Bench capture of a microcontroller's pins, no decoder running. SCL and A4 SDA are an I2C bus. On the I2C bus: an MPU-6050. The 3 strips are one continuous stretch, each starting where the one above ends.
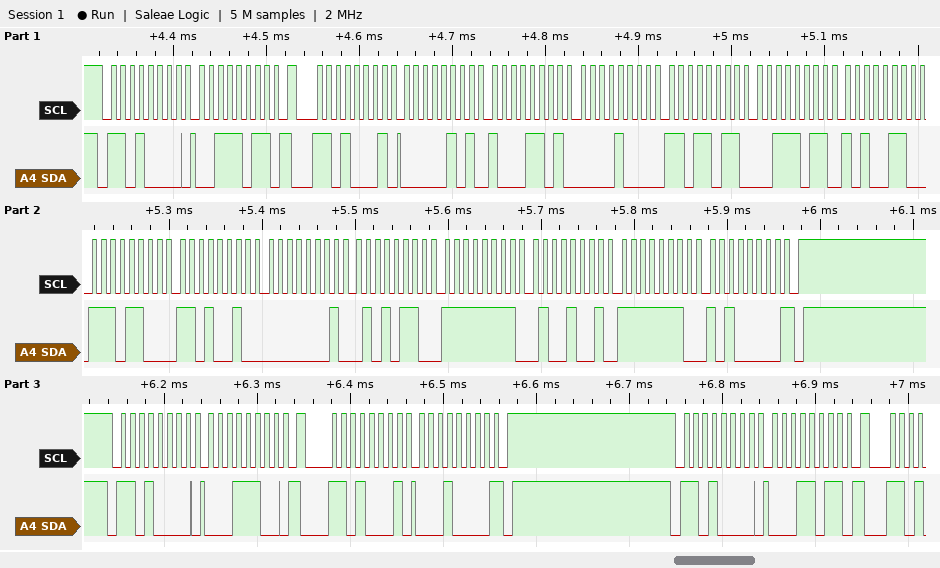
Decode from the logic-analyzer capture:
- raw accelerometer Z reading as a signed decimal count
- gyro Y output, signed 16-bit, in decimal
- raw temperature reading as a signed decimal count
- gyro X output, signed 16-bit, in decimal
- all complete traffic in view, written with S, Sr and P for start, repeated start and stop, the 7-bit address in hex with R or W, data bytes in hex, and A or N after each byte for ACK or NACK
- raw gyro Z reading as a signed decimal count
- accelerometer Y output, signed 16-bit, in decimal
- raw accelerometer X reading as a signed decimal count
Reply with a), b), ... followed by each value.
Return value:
a) 15270
b) -183
c) -4910
d) 342
e) S 68W A 3B A Sr 68R A 05 A 8D A 08 A DB A 3B A A6 A EC A D2 A 01 A 56 A FF A 49 A FE A A0 N P S 68W A 1C A Sr 68R A 10 N P S 68W A 1B A
f) -352
g) 2267
h) 1421
